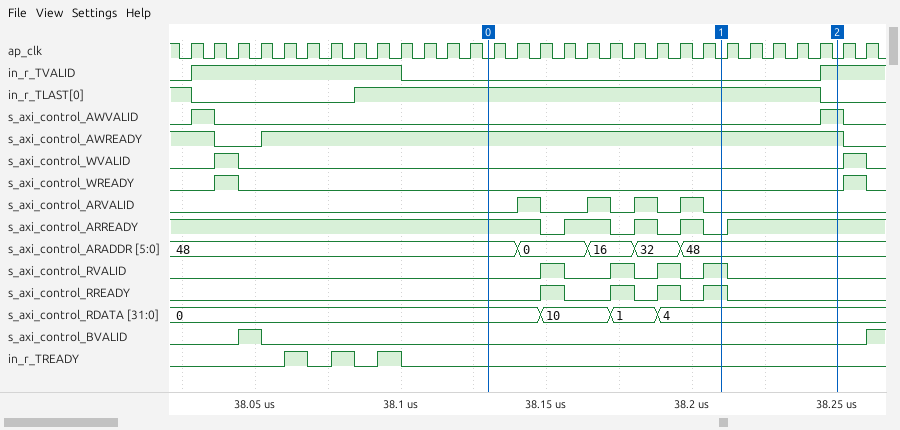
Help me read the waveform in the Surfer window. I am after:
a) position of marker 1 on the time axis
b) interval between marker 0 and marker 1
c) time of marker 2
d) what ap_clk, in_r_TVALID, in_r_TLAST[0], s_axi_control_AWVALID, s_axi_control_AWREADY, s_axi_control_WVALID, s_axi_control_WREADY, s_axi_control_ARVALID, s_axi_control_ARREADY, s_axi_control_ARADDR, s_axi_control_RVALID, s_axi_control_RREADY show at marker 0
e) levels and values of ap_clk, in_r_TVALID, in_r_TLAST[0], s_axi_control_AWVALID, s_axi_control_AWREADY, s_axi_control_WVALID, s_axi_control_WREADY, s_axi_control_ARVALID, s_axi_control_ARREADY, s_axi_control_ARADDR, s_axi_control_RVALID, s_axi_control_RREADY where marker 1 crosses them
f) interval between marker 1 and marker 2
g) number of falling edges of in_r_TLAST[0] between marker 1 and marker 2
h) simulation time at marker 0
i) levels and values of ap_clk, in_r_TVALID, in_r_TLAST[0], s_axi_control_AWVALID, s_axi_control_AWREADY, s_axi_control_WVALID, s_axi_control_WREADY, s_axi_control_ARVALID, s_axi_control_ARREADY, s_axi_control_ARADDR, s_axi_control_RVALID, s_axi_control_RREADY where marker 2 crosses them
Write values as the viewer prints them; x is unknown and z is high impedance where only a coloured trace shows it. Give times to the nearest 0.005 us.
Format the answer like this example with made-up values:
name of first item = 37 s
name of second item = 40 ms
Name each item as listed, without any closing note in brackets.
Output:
position of marker 1 on the time axis = 38.21 us
interval between marker 0 and marker 1 = 0.08 us
time of marker 2 = 38.25 us
what ap_clk, in_r_TVALID, in_r_TLAST[0], s_axi_control_AWVALID, s_axi_control_AWREADY, s_axi_control_WVALID, s_axi_control_WREADY, s_axi_control_ARVALID, s_axi_control_ARREADY, s_axi_control_ARADDR, s_axi_control_RVALID, s_axi_control_RREADY show at marker 0 = ap_clk=0, in_r_TVALID=0, in_r_TLAST[0]=1, s_axi_control_AWVALID=0, s_axi_control_AWREADY=1, s_axi_control_WVALID=0, s_axi_control_WREADY=0, s_axi_control_ARVALID=0, s_axi_control_ARREADY=1, s_axi_control_ARADDR=48, s_axi_control_RVALID=0, s_axi_control_RREADY=0
levels and values of ap_clk, in_r_TVALID, in_r_TLAST[0], s_axi_control_AWVALID, s_axi_control_AWREADY, s_axi_control_WVALID, s_axi_control_WREADY, s_axi_control_ARVALID, s_axi_control_ARREADY, s_axi_control_ARADDR, s_axi_control_RVALID, s_axi_control_RREADY where marker 1 crosses them = ap_clk=0, in_r_TVALID=0, in_r_TLAST[0]=1, s_axi_control_AWVALID=0, s_axi_control_AWREADY=1, s_axi_control_WVALID=0, s_axi_control_WREADY=0, s_axi_control_ARVALID=0, s_axi_control_ARREADY=0, s_axi_control_ARADDR=48, s_axi_control_RVALID=1, s_axi_control_RREADY=1
interval between marker 1 and marker 2 = 0.04 us
number of falling edges of in_r_TLAST[0] between marker 1 and marker 2 = 1
simulation time at marker 0 = 38.13 us
levels and values of ap_clk, in_r_TVALID, in_r_TLAST[0], s_axi_control_AWVALID, s_axi_control_AWREADY, s_axi_control_WVALID, s_axi_control_WREADY, s_axi_control_ARVALID, s_axi_control_ARREADY, s_axi_control_ARADDR, s_axi_control_RVALID, s_axi_control_RREADY where marker 2 crosses them = ap_clk=0, in_r_TVALID=1, in_r_TLAST[0]=0, s_axi_control_AWVALID=1, s_axi_control_AWREADY=1, s_axi_control_WVALID=0, s_axi_control_WREADY=0, s_axi_control_ARVALID=0, s_axi_control_ARREADY=1, s_axi_control_ARADDR=48, s_axi_control_RVALID=0, s_axi_control_RREADY=0
